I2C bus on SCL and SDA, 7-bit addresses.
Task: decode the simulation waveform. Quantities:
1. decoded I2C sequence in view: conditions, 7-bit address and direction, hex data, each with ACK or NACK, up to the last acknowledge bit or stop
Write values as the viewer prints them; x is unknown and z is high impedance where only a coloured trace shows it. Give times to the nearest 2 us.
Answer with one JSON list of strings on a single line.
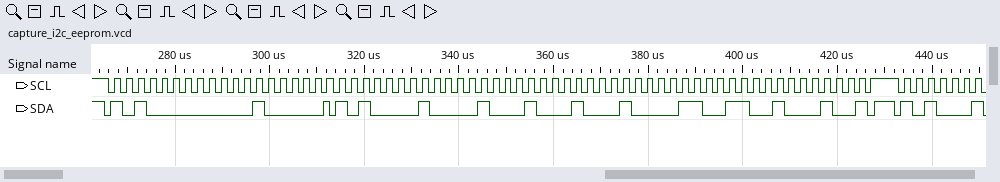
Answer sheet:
["start, address 50 write ACK, 10 ACK, repeated start, address 50 read ACK, 11 ACK, 22 ACK, 33 ACK, 44 NACK, stop"]
